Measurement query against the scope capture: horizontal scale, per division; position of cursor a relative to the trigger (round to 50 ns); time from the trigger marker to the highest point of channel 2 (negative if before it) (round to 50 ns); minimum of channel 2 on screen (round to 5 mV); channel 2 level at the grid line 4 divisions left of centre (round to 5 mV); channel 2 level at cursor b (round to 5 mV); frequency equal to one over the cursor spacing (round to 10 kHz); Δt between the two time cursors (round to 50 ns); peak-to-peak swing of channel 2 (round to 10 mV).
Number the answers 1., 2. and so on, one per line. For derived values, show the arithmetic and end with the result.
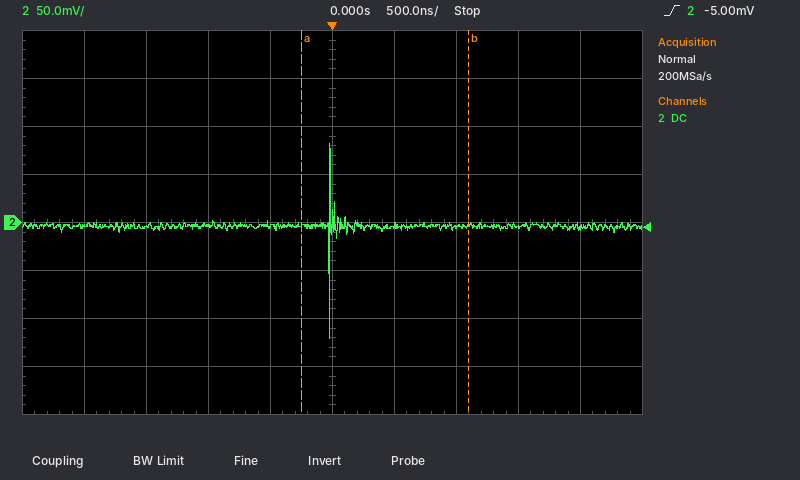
1. 500 ns
2. -250 ns
3. 0 ns
4. -120 mV
5. -5 mV
6. -5 mV
7. 1 / 1.35 µs ≈ 740 kHz
8. 1.35 µs
9. 200 mV
